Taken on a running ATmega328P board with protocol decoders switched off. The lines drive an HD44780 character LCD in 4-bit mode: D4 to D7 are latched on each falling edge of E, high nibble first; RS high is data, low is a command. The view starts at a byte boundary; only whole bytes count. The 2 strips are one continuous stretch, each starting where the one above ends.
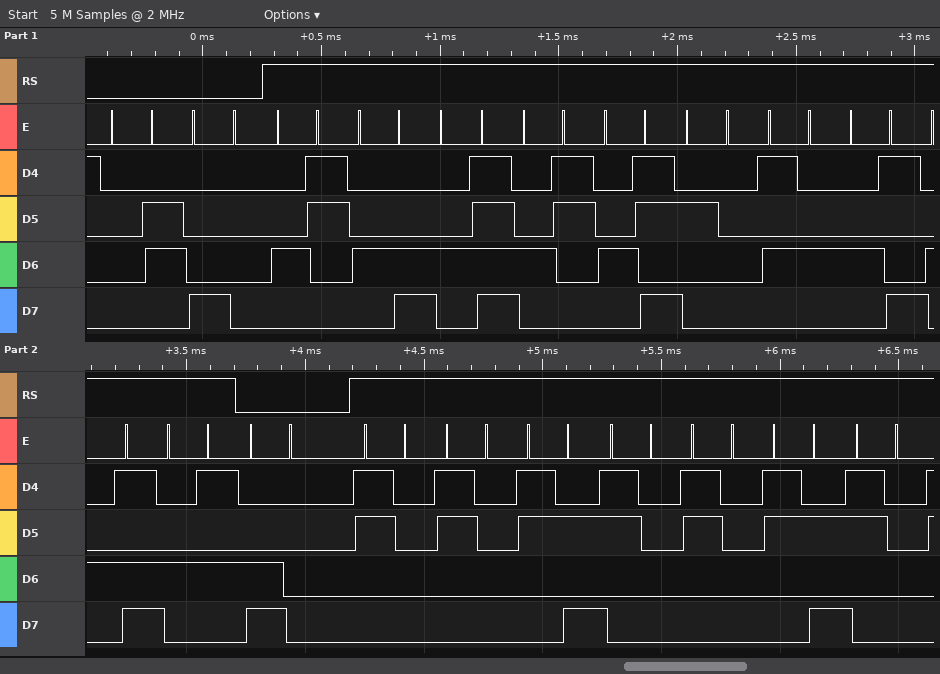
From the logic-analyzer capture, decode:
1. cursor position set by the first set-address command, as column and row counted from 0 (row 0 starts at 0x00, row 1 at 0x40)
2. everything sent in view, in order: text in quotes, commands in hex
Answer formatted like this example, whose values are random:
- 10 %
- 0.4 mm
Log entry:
- column 0, row 0
- 0x06 0x80 "CLOCK TIME" 0xC0 "00:00:0"
